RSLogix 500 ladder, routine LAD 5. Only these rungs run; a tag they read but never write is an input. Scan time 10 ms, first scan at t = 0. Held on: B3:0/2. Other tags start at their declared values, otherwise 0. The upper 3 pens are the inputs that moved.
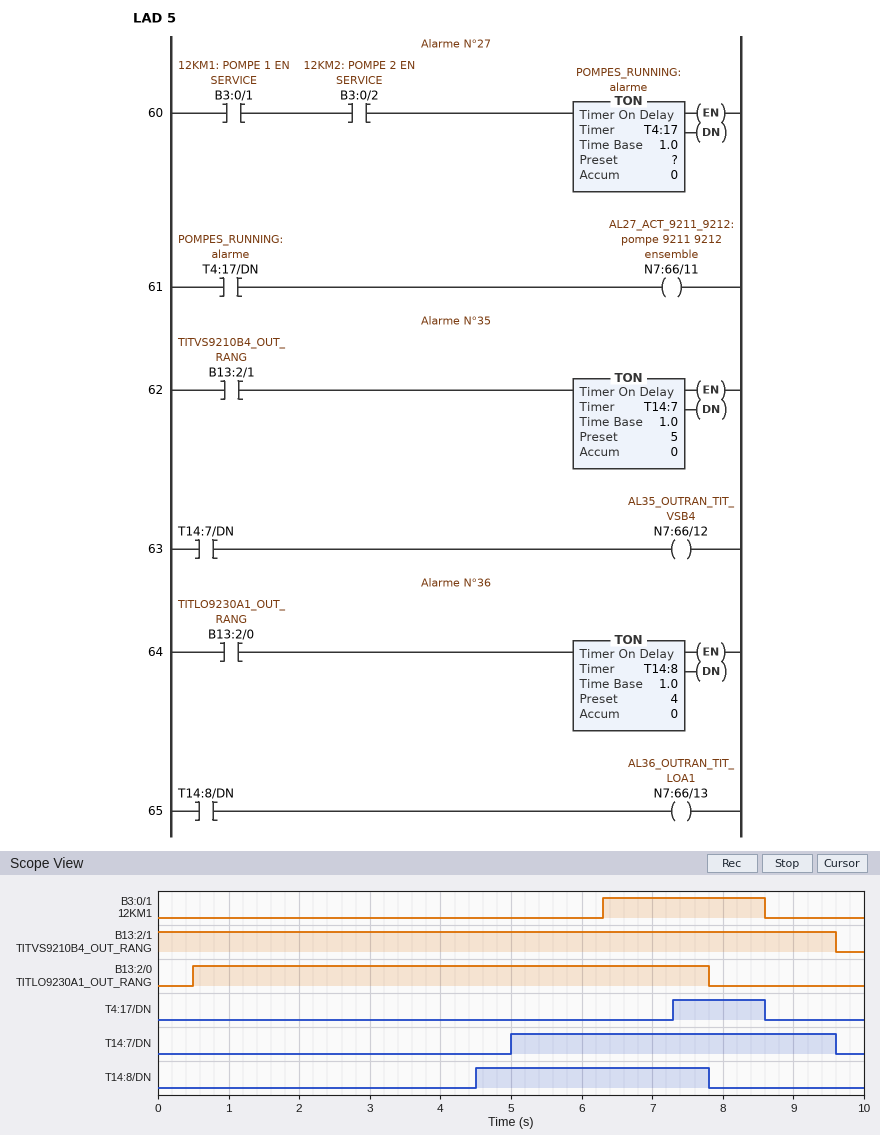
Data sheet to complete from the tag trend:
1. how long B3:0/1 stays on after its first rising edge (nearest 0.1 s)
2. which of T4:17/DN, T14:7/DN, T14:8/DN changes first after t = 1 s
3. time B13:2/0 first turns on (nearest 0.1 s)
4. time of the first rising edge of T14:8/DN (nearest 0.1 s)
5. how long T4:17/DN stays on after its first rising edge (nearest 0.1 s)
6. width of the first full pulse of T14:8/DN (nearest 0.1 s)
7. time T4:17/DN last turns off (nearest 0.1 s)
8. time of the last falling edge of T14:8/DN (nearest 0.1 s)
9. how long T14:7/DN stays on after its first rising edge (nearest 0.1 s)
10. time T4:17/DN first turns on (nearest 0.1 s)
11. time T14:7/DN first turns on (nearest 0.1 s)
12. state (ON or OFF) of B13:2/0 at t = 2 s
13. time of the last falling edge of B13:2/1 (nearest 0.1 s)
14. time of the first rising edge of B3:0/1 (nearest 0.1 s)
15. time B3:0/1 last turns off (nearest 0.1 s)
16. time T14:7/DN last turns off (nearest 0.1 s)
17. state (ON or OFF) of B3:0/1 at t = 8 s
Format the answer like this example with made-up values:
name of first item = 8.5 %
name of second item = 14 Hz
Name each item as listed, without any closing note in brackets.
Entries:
how long B3:0/1 stays on after its first rising edge = 2.3 s
which of T4:17/DN, T14:7/DN, T14:8/DN changes first after t = 1 s = T14:8/DN
time B13:2/0 first turns on = 0.5 s
time of the first rising edge of T14:8/DN = 4.5 s
how long T4:17/DN stays on after its first rising edge = 1.3 s
width of the first full pulse of T14:8/DN = 3.3 s
time T4:17/DN last turns off = 8.6 s
time of the last falling edge of T14:8/DN = 7.8 s
how long T14:7/DN stays on after its first rising edge = 4.6 s
time T4:17/DN first turns on = 7.3 s
time T14:7/DN first turns on = 5.0 s
state (ON or OFF) of B13:2/0 at t = 2 s = ON
time of the last falling edge of B13:2/1 = 9.6 s
time of the first rising edge of B3:0/1 = 6.3 s
time B3:0/1 last turns off = 8.6 s
time T14:7/DN last turns off = 9.6 s
state (ON or OFF) of B3:0/1 at t = 8 s = ON
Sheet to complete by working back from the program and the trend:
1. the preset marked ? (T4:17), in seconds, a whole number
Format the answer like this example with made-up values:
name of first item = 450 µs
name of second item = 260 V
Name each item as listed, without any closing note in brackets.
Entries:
the preset marked ? (T4:17), in seconds, a whole number = 1 s
